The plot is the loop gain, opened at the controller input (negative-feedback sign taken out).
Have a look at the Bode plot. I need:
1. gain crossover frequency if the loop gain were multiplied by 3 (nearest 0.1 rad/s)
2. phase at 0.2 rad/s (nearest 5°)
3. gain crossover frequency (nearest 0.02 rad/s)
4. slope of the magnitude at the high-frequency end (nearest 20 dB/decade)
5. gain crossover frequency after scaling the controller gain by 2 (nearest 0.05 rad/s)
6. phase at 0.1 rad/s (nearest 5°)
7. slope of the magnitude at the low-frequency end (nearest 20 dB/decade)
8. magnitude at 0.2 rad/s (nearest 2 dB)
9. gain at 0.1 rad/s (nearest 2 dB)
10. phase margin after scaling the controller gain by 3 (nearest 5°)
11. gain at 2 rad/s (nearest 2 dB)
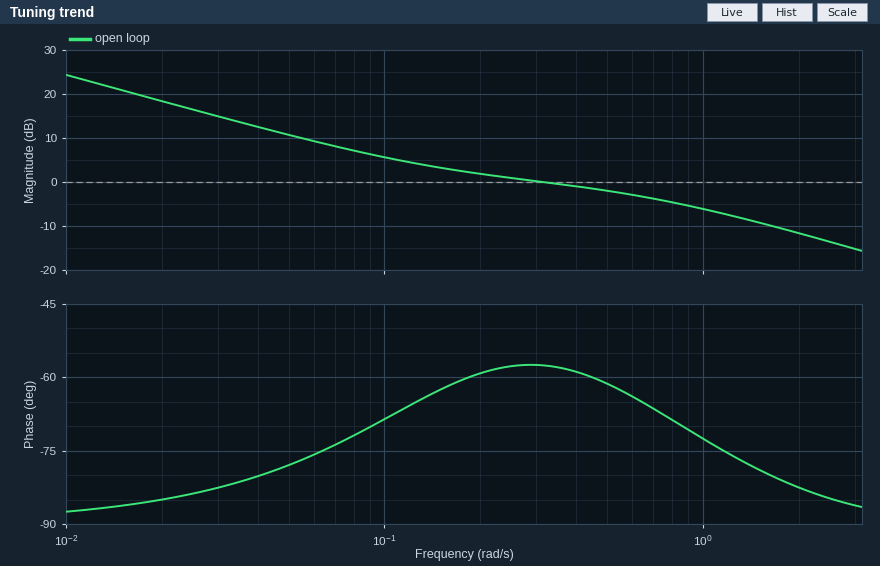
1.6 rad/s
-60°
0.32 rad/s
-20 dB/decade
1.00 rad/s
-70°
-20 dB/decade
2 dB
6 dB
100°
-12 dB
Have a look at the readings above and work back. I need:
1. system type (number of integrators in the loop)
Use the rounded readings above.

1
